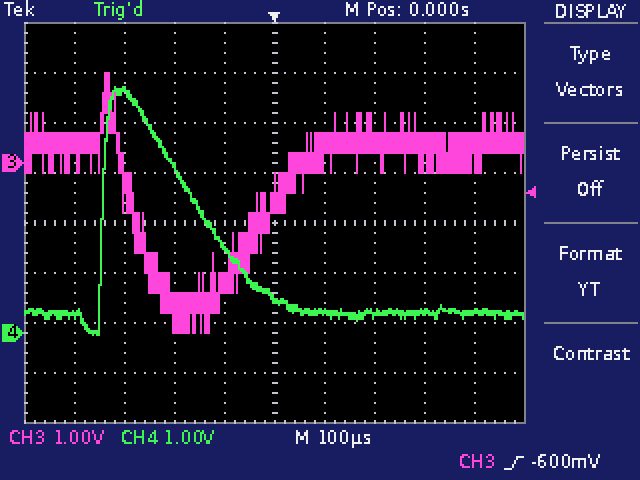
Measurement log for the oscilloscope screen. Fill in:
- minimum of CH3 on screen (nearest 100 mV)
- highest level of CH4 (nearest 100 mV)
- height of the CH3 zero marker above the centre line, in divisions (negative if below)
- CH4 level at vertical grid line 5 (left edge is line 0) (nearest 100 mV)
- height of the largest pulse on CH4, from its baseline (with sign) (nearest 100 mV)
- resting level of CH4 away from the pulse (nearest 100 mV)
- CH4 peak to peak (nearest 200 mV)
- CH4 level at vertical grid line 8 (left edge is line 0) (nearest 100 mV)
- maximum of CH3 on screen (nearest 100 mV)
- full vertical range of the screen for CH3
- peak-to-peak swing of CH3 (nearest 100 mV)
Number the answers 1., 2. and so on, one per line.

1. -3.4 V
2. 4.9 V
3. +1.2 div
4. 700 mV
5. +4.5 V
6. 400 mV
7. 5.0 V
8. 400 mV
9. 1.8 V
10. 8 V
11. 5.2 V
